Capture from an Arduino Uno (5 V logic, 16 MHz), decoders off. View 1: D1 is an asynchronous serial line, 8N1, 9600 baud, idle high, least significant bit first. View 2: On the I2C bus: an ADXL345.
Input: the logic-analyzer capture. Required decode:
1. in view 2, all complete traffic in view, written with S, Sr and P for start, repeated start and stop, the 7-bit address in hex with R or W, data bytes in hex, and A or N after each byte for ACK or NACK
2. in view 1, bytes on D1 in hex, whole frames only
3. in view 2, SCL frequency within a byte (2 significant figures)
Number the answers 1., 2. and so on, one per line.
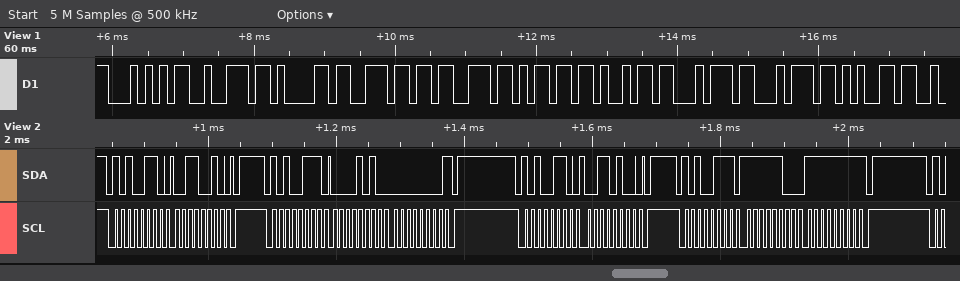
1. S 53W A 32 A P S 53R A 0A A 00 N P S 53W A 34 A P S 53R A FC A FF N P
2. 54 72 61 6E 73 6D 69 74 74 65
3. 100 kHz
